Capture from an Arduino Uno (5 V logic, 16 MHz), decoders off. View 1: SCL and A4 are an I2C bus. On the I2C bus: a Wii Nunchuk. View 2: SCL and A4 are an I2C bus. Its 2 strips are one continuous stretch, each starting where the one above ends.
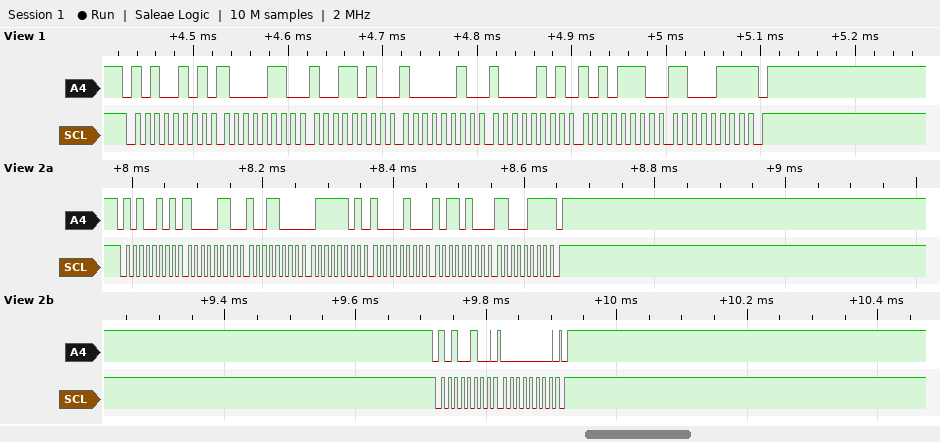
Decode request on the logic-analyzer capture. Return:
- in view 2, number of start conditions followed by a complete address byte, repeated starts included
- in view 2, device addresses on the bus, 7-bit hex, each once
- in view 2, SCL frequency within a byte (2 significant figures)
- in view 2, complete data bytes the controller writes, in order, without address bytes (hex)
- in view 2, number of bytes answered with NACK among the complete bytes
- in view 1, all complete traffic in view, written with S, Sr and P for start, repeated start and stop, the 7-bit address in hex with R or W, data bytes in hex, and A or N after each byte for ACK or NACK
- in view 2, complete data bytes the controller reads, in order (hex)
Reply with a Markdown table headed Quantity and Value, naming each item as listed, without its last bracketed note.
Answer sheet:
| Quantity | Value |
|---|---|
| in view 2, number of start conditions followed by a complete address byte, repeated starts included | 2 |
| in view 2, device addresses on the bus, 7-bit hex, each once | 0x52 |
| in view 2, SCL frequency within a byte | 100 kHz |
| in view 2, complete data bytes the controller writes, in order, without address bytes | 00 |
| in view 2, number of bytes answered with NACK among the complete bytes | 1 |
| in view 1, all complete traffic in view, written with S, Sr and P for start, repeated start and stop, the 7-bit address in hex with R or W, data bytes in hex, and A or N after each byte for ACK or NACK | S 52R A 86 A 9A A 82 A 85 A AE A C7 N P |
| in view 2, complete data bytes the controller reads, in order | 86 98 7D 84 B4 C7 |
